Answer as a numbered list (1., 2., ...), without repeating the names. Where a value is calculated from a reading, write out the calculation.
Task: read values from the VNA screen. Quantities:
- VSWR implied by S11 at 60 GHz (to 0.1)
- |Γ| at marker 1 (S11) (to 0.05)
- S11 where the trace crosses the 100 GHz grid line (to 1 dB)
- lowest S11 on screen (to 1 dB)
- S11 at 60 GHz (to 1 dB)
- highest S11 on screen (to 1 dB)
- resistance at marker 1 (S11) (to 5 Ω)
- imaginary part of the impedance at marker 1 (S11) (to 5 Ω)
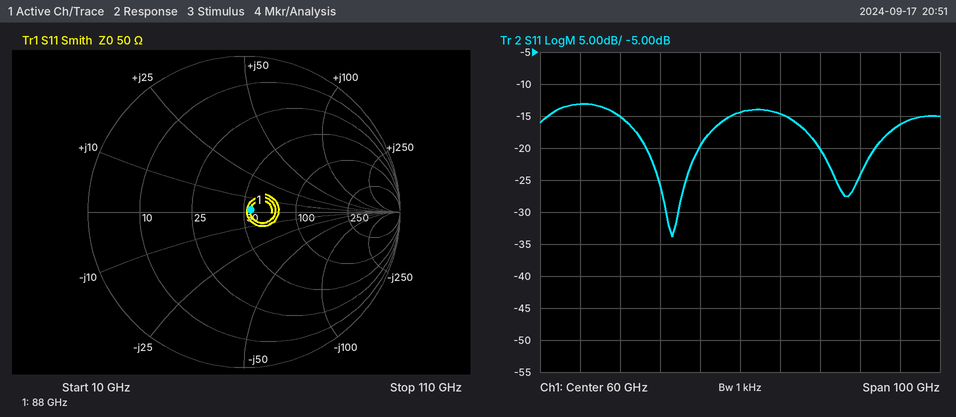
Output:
1. |Γ| = 10^(-14/20) = 0.1995; VSWR = (1 + 0.1995)/(1 − 0.1995) ≈ 1.5
2. 0.05
3. -16 dB
4. -34 dB
5. -14 dB
6. -13 dB
7. 55 Ω
8. 0 Ω
